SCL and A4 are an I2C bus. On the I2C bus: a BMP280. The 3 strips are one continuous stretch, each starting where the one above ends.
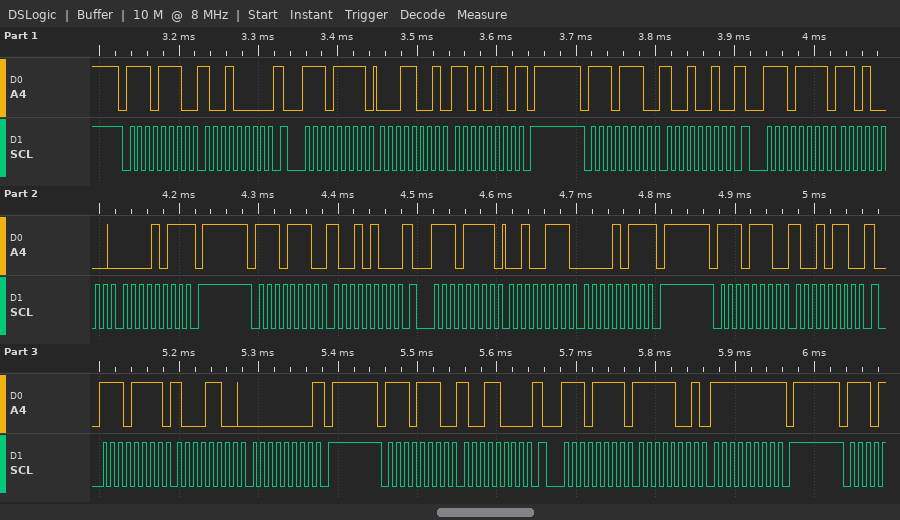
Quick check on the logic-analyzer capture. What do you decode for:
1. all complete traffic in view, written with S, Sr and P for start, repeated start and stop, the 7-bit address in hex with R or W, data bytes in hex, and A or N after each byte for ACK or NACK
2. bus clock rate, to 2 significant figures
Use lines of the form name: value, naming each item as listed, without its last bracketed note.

all complete traffic in view, written with S, Sr and P for start, repeated start and stop, the 7-bit address in hex with R or W, data bytes in hex, and A or N after each byte for ACK or NACK: S 77W A 90 A Sr 77R A 19 A D6 N P S 77W A 92 A Sr 77R A D0 A 0B N P S 77W A 94 A Sr 77R A 27 A 0B N P S 77W A 96 A Sr 77R A 8C A 00 N P S 77W A 98 A Sr 77R A F9 A FF N P
bus clock rate, to 2 significant figures: 100 kHz
